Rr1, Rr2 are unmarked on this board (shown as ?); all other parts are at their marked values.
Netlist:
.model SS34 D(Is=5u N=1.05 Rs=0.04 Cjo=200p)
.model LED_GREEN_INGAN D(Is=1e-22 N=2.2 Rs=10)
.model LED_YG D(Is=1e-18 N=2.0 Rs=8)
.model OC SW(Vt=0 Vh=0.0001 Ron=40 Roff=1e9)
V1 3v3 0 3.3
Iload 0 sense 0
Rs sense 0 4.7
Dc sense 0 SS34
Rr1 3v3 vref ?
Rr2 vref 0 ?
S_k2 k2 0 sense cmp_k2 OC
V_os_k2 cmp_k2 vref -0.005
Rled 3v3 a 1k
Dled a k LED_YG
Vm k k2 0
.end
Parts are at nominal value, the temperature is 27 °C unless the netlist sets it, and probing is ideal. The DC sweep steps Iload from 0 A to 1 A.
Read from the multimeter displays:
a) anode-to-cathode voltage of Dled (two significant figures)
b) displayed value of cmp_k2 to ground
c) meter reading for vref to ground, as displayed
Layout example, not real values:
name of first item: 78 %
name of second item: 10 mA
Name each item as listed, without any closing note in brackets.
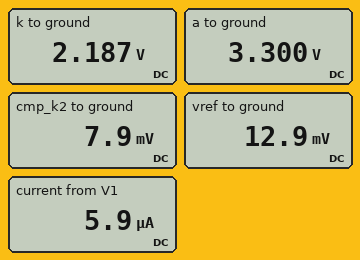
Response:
anode-to-cathode voltage of Dled: 1.1 V
displayed value of cmp_k2 to ground: 7.9 mV
meter reading for vref to ground, as displayed: 12.9 mV
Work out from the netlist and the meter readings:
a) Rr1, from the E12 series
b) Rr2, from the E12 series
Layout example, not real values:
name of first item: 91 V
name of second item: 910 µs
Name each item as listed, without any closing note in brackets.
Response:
Rr1, from the E12 series: 560 kΩ
Rr2, from the E12 series: 2.2 kΩ
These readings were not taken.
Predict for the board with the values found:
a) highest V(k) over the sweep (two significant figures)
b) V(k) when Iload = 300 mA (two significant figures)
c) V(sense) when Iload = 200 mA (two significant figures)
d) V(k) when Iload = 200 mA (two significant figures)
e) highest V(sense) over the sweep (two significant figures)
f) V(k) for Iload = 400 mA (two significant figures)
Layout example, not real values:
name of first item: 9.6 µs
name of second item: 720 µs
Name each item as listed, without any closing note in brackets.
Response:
highest V(k) over the sweep: 2.2 V
V(k) when Iload = 300 mA: 57 mV
V(sense) when Iload = 200 mA: 280 mV
V(k) when Iload = 200 mA: 57 mV
highest V(sense) over the sweep: 370 mV
V(k) for Iload = 400 mA: 57 mV
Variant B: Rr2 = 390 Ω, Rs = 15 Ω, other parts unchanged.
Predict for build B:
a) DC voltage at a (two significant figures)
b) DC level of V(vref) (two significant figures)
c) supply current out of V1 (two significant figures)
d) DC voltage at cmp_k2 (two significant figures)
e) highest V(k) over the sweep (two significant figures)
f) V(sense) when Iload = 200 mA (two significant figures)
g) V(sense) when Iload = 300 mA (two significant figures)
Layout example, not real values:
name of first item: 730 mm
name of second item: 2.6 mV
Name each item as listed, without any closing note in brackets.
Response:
DC voltage at a: 1.9 V
DC level of V(vref): 2.3 mV
supply current out of V1: 1.4 mA
DC voltage at cmp_k2: -2.7 mV
highest V(k) over the sweep: 57 mV
V(sense) when Iload = 200 mA: 290 mV
V(sense) when Iload = 300 mA: 310 mV
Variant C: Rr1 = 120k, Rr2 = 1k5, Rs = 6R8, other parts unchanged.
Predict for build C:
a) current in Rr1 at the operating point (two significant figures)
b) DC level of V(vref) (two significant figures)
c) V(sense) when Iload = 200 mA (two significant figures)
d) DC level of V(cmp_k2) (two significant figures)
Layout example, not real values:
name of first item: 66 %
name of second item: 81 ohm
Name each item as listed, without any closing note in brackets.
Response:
current in Rr1 at the operating point: 27 µA
DC level of V(vref): 41 mV
V(sense) when Iload = 200 mA: 290 mV
DC level of V(cmp_k2): 36 mV
